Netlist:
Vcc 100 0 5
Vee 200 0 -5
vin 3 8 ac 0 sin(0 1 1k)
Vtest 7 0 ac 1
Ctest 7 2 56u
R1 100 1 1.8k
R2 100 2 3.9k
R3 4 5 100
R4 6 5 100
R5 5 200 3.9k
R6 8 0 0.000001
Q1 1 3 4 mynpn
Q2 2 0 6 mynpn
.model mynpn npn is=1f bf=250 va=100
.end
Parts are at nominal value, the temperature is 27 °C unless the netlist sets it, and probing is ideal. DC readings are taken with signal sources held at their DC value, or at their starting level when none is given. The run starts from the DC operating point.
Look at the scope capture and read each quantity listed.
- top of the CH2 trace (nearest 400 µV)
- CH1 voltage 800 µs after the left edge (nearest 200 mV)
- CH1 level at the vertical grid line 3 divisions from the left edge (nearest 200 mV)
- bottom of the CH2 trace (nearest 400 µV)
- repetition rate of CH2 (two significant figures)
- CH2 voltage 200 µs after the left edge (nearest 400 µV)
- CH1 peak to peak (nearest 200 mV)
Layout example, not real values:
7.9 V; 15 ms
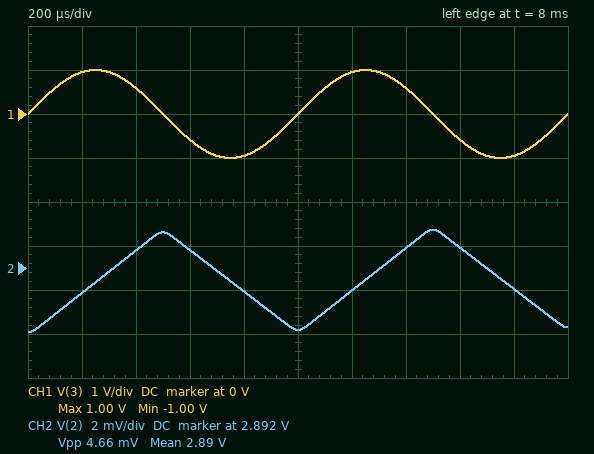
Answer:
2.8936 V; -1.0 V; -600 mV; 2.8892 V; 1.0 kHz; 2.8908 V; 2.0 V
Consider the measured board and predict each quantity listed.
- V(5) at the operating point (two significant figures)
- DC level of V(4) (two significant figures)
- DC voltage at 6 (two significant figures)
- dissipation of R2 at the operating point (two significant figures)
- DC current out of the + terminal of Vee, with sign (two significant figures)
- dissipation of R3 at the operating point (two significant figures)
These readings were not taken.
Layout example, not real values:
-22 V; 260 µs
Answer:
-750 mV; -700 mV; -700 mV; 1.1 mW; -1.1 mA; 30 µW
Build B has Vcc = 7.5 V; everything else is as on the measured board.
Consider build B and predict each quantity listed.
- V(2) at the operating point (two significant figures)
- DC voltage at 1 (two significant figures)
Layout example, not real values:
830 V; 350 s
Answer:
5.4 V; 6.5 V
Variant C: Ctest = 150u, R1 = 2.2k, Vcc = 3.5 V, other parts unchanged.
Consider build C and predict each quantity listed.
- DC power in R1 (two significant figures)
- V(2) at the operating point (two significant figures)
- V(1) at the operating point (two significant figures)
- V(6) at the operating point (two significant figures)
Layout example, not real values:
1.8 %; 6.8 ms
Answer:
650 µW; 1.4 V; 2.3 V; -700 mV
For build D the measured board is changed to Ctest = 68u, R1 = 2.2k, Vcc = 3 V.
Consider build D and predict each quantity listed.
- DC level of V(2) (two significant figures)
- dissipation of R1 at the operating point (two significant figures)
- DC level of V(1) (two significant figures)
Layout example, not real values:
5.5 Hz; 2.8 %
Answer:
890 mV; 650 µW; 1.8 V
